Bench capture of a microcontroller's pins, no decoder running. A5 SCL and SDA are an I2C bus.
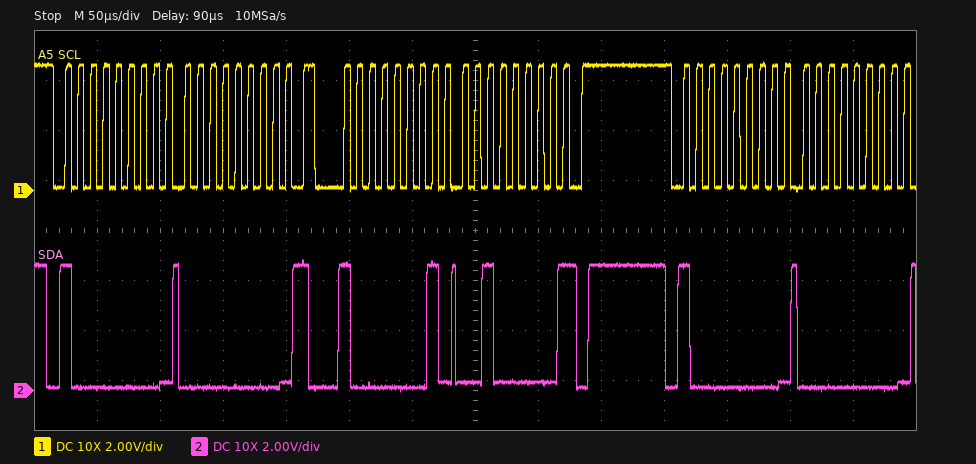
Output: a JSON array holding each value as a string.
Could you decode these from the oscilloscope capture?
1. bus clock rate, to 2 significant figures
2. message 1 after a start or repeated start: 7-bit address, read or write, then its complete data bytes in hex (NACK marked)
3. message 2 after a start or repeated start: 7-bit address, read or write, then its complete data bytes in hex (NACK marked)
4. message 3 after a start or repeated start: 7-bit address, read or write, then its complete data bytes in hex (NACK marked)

["100 kHz", "0x40 write: 00", "0x40 read: 20 NACK", "0x40 write: 00"]
